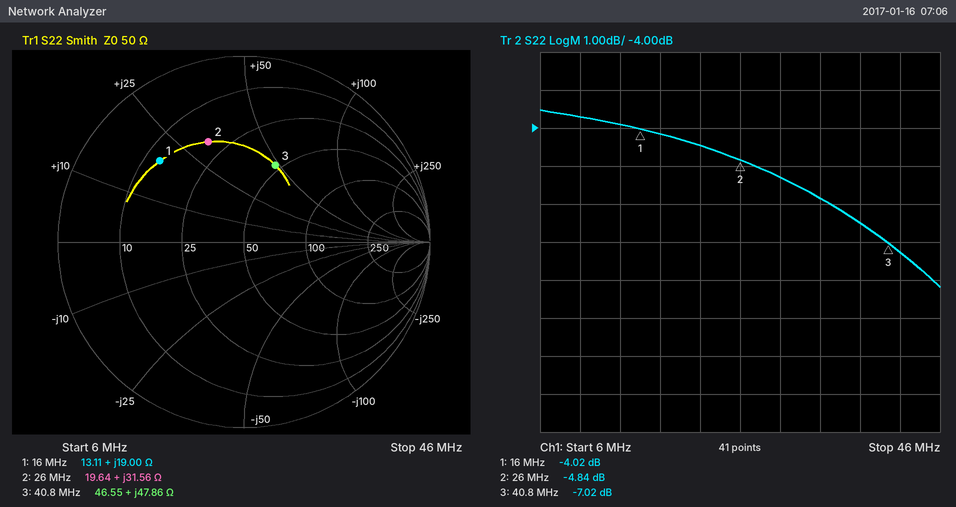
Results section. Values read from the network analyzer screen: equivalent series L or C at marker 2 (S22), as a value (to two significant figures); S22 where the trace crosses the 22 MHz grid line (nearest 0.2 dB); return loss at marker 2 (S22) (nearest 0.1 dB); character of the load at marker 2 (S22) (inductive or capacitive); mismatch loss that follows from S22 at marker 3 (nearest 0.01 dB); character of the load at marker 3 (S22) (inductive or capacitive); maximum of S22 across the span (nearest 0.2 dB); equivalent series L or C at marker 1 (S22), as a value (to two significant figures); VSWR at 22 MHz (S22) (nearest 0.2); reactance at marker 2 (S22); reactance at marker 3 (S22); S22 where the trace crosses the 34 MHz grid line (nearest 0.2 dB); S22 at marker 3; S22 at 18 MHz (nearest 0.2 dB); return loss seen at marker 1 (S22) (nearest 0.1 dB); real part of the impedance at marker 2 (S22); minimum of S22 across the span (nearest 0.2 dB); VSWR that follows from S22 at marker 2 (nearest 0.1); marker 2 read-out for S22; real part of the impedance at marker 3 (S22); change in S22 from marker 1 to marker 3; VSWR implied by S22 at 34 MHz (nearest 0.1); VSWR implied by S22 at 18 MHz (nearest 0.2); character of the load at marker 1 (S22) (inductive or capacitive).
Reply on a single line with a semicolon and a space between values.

190 nH; -4.4 dB; 4.8 dB; inductive; 0.96 dB; inductive; -3.6 dB; 190 nH; 4.0; +31.56 Ω; +47.86 Ω; -5.8 dB; -7.02 dB; -4.2 dB; 4.0 dB; 19.64 Ω; -8.2 dB; 3.7; -4.84 dB; 46.55 Ω; -3.00 dB; 3.1; 4.2; inductive
